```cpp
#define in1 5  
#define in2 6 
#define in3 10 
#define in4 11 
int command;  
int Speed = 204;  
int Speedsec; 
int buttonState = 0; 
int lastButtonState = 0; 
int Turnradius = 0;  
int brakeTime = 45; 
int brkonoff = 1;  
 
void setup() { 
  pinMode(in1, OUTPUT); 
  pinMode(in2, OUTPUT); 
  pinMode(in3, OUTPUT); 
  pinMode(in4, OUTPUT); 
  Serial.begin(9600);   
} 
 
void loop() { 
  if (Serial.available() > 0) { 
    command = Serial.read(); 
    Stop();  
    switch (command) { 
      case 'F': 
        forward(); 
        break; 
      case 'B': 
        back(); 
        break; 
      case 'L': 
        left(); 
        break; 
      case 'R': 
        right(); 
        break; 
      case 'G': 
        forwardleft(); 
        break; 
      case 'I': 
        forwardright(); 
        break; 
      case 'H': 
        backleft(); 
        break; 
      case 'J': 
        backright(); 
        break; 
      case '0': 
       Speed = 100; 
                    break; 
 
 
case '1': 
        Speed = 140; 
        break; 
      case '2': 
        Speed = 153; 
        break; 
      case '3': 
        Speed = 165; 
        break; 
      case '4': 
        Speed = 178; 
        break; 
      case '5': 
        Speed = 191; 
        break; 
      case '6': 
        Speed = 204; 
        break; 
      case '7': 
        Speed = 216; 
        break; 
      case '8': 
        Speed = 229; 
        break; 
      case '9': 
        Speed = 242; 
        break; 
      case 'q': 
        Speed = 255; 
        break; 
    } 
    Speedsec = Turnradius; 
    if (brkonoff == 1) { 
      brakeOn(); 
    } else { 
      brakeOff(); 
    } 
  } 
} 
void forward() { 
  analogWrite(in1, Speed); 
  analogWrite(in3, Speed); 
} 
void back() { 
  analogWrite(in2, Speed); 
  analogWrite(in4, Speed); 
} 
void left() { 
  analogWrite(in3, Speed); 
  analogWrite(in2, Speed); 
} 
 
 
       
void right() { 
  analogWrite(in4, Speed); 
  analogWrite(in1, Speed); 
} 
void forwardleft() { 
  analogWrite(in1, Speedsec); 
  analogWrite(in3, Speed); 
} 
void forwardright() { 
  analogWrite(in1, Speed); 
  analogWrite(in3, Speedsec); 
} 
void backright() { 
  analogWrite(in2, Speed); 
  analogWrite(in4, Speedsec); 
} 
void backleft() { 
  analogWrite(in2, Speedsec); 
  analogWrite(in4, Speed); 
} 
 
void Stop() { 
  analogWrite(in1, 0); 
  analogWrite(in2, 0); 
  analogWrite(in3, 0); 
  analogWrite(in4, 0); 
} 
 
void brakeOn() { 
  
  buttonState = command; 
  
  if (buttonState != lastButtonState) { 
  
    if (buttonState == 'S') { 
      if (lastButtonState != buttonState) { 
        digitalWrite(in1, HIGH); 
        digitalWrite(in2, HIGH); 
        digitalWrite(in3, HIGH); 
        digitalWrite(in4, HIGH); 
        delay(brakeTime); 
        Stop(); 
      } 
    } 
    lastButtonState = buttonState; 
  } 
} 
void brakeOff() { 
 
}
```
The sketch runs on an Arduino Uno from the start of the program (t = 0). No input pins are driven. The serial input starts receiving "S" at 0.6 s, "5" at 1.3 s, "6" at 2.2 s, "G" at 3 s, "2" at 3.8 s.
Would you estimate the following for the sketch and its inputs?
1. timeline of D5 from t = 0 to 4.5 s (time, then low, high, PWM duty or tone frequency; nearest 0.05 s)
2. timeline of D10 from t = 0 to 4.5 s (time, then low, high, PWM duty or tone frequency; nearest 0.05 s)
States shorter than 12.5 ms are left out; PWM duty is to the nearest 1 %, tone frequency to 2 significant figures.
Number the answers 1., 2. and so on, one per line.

1. 0 s low; 0.6 s high; 0.65 s low
2. 0 s low; 0.6 s high; 0.65 s low; 3 s PWM 80 %; 3.8 s low
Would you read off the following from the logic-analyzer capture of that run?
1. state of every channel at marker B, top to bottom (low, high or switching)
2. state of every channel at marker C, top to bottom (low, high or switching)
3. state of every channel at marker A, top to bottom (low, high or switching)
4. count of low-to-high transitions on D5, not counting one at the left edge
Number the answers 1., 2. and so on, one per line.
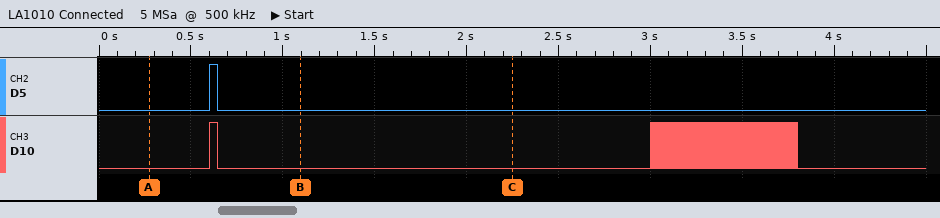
1. D5 low, D10 low
2. D5 low, D10 low
3. D5 low, D10 low
4. 1
